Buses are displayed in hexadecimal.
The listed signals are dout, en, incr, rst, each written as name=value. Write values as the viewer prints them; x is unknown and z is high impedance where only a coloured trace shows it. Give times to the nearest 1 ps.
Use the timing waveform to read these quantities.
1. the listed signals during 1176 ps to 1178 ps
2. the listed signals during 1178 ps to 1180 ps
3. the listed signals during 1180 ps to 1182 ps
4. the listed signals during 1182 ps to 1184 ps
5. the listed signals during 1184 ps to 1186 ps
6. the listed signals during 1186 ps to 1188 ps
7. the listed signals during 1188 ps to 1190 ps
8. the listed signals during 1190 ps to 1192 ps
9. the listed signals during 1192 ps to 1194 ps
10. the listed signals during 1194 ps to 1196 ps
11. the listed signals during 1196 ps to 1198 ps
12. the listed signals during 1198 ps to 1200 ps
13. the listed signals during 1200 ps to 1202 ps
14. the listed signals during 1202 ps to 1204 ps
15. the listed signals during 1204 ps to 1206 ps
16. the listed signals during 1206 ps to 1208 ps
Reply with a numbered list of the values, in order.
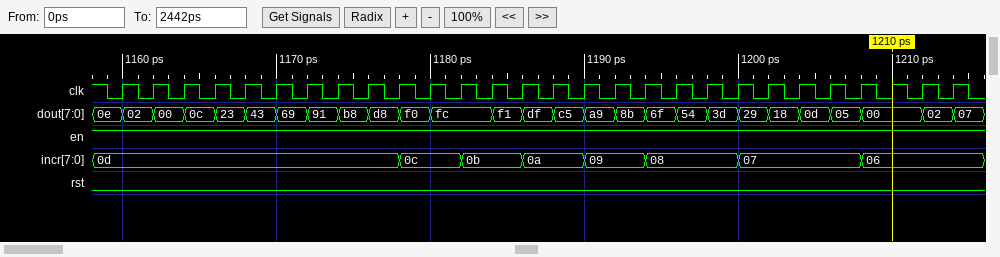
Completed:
1. dout=d8, en=1, incr=0d, rst=0
2. dout=f0, en=1, incr=0c, rst=0
3. dout=fc, en=1, incr=0c, rst=0
4. dout=fc, en=1, incr=0b, rst=0
5. dout=f1, en=1, incr=0b, rst=0
6. dout=df, en=1, incr=0a, rst=0
7. dout=c5, en=1, incr=0a, rst=0
8. dout=a9, en=1, incr=09, rst=0
9. dout=8b, en=1, incr=09, rst=0
10. dout=6f, en=1, incr=08, rst=0
11. dout=54, en=1, incr=08, rst=0
12. dout=3d, en=1, incr=08, rst=0
13. dout=29, en=1, incr=07, rst=0
14. dout=18, en=1, incr=07, rst=0
15. dout=0d, en=1, incr=07, rst=0
16. dout=05, en=1, incr=07, rst=0
